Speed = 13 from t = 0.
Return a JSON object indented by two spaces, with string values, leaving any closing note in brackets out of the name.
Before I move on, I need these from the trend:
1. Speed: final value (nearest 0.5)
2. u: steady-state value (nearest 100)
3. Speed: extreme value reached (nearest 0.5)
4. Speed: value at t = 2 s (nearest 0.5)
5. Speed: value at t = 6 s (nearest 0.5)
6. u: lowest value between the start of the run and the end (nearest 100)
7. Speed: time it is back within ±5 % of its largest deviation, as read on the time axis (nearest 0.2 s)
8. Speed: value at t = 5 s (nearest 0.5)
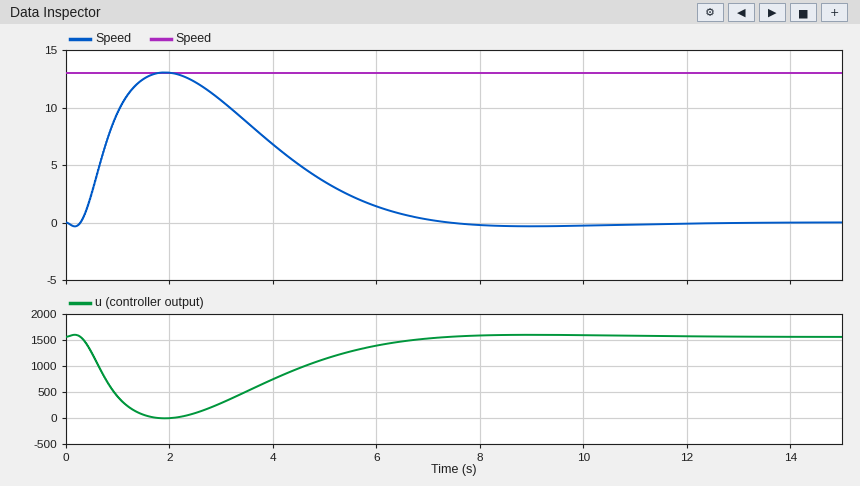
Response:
{
  "Speed: final value": "0.0",
  "u: steady-state value": "1600",
  "Speed: extreme value reached": "13.0",
  "Speed: value at t = 2 s": "13.0",
  "Speed: value at t = 6 s": "1.5",
  "u: lowest value between the start of the run and the end": "0",
  "Speed: time it is back within ±5 % of its largest deviation, as read on the time axis": "6.6 s",
  "Speed: value at t = 5 s": "3.5"
}
